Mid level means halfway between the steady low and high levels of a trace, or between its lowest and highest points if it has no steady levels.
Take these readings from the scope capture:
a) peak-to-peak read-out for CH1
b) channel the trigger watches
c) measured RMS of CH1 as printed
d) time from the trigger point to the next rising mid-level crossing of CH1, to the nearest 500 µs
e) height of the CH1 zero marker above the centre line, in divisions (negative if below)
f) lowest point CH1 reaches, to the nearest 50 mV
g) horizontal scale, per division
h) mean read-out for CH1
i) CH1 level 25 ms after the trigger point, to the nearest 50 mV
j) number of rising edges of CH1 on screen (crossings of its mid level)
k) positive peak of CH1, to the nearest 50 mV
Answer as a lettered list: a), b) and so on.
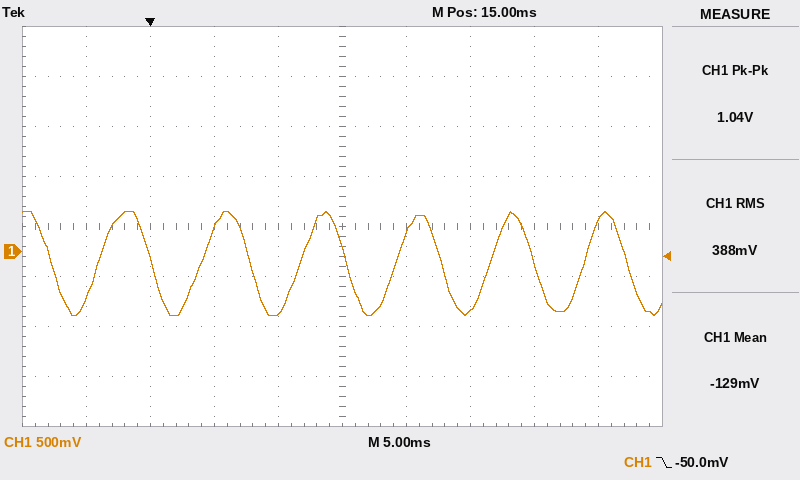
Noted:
a) 1.04 V
b) CH1
c) 388 mV
d) 4.0 ms
e) -0.5 div
f) -650 mV
g) 5 ms
h) -129 mV
i) -600 mV
j) 6
k) 400 mV
